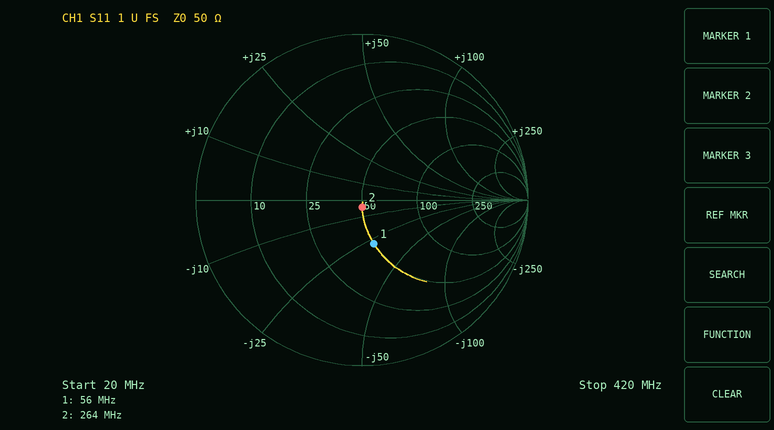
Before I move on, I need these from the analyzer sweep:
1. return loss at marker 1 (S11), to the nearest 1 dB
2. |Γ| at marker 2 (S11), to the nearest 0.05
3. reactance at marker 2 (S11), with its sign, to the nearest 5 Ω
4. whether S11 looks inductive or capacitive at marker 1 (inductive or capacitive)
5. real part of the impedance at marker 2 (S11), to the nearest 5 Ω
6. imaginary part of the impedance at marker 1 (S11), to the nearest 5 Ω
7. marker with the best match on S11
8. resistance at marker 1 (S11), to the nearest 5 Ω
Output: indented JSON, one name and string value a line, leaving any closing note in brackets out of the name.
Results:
{
  "return loss at marker 1 (S11), to the nearest 1 dB": "11 dB",
  "|Γ| at marker 2 (S11), to the nearest 0.05": "0.05",
  "reactance at marker 2 (S11), with its sign, to the nearest 5 Ω": "-5 Ω",
  "whether S11 looks inductive or capacitive at marker 1": "capacitive",
  "real part of the impedance at marker 2 (S11), to the nearest 5 Ω": "50 Ω",
  "imaginary part of the impedance at marker 1 (S11), to the nearest 5 Ω": "-30 Ω",
  "marker with the best match on S11": "marker 2",
  "resistance at marker 1 (S11), to the nearest 5 Ω": "50 Ω"
}
